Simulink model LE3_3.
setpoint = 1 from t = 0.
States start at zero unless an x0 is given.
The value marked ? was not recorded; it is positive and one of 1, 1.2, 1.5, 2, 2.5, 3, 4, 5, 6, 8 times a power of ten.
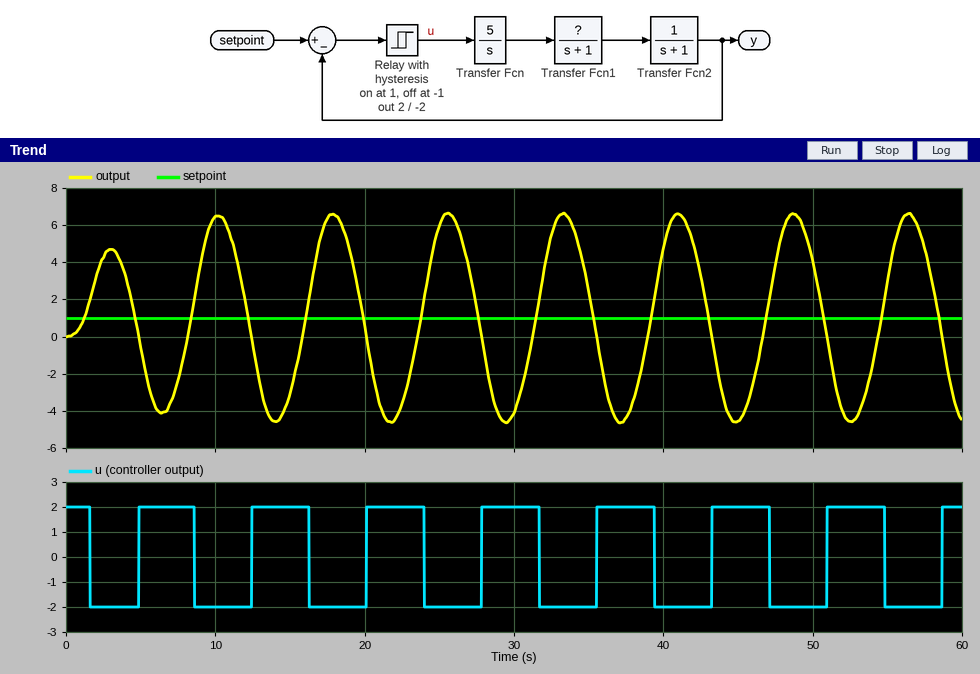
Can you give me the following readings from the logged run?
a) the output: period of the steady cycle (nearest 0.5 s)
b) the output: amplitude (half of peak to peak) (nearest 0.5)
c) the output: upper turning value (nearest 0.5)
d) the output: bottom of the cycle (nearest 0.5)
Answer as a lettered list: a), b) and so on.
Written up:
a) 7.5 s
b) 5.5
c) 6.5
d) -4.5
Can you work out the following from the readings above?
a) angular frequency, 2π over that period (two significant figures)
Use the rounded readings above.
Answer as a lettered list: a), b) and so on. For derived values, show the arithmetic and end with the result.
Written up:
a) 2π / 7.5 = 0.84 rad/s
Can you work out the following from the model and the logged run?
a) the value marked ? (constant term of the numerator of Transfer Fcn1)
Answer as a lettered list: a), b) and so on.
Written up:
a) 0.6
